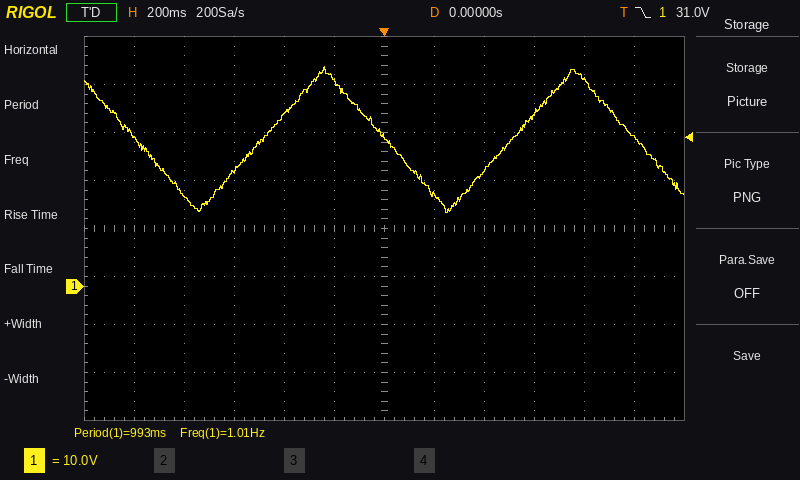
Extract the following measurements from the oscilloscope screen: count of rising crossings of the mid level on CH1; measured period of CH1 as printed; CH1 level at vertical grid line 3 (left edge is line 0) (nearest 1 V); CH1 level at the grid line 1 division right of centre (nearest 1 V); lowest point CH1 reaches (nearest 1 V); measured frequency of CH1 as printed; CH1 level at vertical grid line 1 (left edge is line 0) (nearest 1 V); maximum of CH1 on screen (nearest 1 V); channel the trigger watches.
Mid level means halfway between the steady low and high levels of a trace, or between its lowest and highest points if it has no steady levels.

2
993 ms
24 V
19 V
15 V
1.01 Hz
31 V
46 V
CH1
